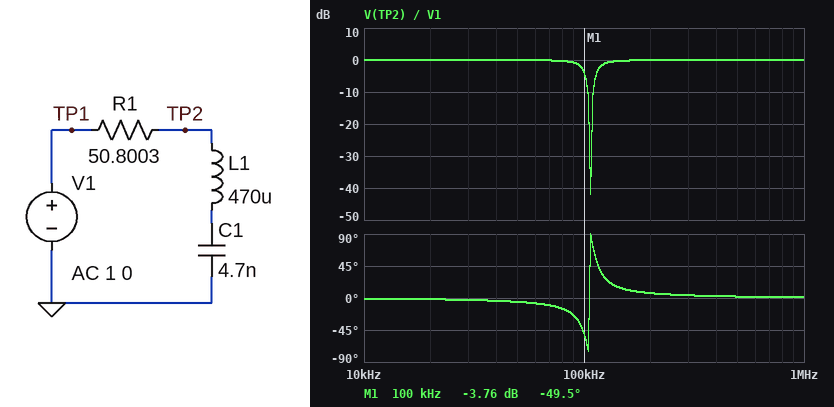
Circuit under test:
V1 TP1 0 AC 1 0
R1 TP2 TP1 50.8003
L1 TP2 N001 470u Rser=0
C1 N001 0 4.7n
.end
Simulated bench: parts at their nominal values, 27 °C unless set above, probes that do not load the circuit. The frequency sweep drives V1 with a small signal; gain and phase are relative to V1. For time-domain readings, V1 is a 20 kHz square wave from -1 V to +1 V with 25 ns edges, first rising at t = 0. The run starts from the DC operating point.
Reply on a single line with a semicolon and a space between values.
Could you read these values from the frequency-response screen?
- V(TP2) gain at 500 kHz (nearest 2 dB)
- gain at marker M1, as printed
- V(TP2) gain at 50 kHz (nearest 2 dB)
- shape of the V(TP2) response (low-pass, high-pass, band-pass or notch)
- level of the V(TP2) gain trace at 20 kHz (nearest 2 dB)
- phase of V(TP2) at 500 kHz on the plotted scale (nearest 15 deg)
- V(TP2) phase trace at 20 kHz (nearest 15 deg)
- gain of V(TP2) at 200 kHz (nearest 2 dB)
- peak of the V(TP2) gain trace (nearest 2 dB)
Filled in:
0 dB; -3.76 dB; 0 dB; notch; 0 dB; 0 deg; 0 deg; 0 dB; 0 dB
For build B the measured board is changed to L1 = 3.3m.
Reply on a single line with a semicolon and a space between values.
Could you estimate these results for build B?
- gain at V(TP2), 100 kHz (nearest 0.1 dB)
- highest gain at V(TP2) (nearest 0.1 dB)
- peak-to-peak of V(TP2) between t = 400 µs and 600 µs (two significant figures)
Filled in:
0 dB; 0 dB; 2.1 V
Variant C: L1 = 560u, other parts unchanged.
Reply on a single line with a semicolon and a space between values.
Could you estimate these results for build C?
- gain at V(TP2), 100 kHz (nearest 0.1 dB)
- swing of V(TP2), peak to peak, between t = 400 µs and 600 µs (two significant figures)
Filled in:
-12.0 dB; 2.6 V
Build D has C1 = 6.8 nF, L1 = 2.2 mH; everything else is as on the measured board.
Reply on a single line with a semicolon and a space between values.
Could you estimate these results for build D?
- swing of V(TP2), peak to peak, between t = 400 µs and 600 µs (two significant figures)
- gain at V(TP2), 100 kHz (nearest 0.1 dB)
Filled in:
2.2 V; 0 dB
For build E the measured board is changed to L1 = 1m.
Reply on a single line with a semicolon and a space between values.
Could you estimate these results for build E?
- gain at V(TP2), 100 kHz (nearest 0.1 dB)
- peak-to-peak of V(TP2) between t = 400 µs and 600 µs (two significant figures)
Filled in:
-0.1 dB; 2.3 V
